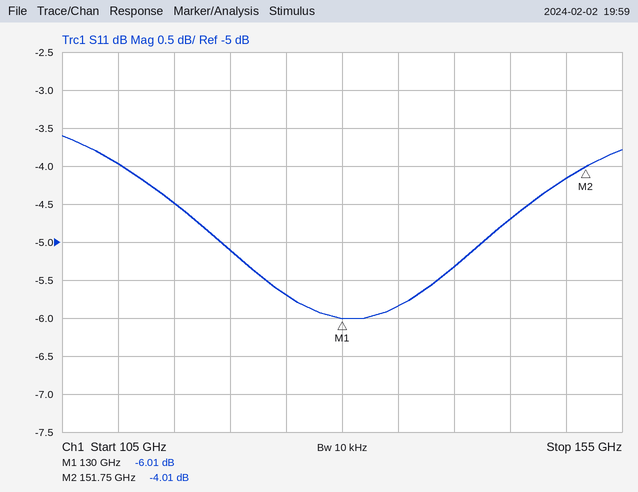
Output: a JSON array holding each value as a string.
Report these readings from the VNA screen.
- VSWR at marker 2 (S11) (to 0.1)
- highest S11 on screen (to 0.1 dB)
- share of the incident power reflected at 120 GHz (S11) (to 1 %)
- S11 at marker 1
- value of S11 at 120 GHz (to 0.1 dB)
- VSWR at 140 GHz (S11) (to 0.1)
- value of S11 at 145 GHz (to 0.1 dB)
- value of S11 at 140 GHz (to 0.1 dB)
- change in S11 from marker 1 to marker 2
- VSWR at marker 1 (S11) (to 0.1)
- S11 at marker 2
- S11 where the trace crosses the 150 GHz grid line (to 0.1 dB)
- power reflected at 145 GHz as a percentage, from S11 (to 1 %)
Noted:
["4.4", "-3.6 dB", "31 %", "-6.01 dB", "-5.1 dB", "3.4", "-4.7 dB", "-5.3 dB", "2.00 dB", "3.0", "-4.01 dB", "-4.2 dB", "34 %"]
